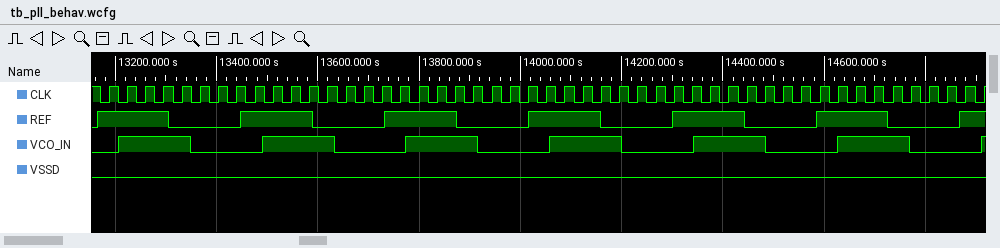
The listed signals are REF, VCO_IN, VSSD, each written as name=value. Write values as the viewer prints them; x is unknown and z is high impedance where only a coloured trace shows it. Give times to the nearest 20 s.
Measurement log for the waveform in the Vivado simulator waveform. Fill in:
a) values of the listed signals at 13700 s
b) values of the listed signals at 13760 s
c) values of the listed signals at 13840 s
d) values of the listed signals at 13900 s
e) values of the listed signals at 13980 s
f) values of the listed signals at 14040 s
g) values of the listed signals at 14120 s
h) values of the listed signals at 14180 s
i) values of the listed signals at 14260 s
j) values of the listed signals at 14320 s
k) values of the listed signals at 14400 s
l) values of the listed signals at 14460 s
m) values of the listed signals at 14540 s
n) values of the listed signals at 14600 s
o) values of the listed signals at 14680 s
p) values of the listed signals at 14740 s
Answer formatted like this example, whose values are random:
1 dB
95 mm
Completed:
REF=0, VCO_IN=0, VSSD=0
REF=1, VCO_IN=0, VSSD=0
REF=1, VCO_IN=1, VSSD=0
REF=0, VCO_IN=1, VSSD=0
REF=0, VCO_IN=0, VSSD=0
REF=1, VCO_IN=0, VSSD=0
REF=1, VCO_IN=1, VSSD=0
REF=0, VCO_IN=1, VSSD=0
REF=0, VCO_IN=0, VSSD=0
REF=1, VCO_IN=0, VSSD=0
REF=1, VCO_IN=1, VSSD=0
REF=0, VCO_IN=1, VSSD=0
REF=0, VCO_IN=0, VSSD=0
REF=1, VCO_IN=0, VSSD=0
REF=1, VCO_IN=1, VSSD=0
REF=0, VCO_IN=1, VSSD=0
